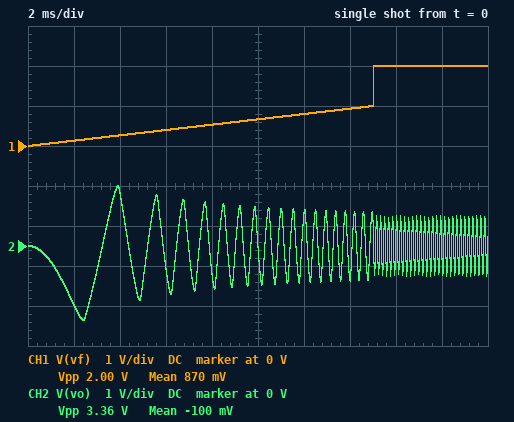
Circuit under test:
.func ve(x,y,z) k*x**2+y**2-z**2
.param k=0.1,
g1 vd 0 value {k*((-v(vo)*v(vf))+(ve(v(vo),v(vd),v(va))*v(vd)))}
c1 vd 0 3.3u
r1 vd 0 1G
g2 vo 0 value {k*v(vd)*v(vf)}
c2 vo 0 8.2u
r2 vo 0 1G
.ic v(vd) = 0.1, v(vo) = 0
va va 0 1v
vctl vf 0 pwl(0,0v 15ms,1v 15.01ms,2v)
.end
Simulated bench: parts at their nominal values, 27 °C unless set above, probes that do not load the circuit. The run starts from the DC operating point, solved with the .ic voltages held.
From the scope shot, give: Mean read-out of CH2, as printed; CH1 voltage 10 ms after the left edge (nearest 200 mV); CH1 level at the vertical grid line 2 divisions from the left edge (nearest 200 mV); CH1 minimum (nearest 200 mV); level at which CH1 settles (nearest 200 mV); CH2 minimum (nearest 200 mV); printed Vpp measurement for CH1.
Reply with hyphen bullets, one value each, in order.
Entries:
- -100 mV
- 600 mV
- 200 mV
- 0 V
- 2.0 V
- -1.8 V
- 2.00 V
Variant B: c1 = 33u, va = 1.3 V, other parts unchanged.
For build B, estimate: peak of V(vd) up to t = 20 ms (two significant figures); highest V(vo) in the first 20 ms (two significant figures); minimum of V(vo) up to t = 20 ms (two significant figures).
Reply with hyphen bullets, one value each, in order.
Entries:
- 1.4 V
- 3.2 V
- -3.4 V
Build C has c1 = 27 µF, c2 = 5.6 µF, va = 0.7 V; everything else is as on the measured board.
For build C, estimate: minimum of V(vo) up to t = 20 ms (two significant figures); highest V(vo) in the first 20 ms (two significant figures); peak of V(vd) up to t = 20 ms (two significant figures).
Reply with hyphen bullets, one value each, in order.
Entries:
- -1.7 V
- 1.7 V
- 750 mV
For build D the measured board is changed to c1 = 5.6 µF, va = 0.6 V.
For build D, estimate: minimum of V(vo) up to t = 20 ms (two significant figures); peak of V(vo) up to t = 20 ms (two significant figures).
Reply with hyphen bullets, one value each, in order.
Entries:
- -870 mV
- 700 mV
